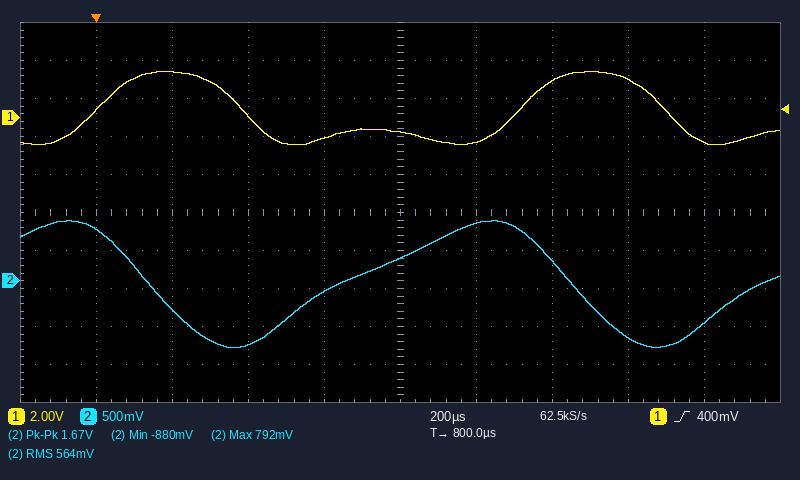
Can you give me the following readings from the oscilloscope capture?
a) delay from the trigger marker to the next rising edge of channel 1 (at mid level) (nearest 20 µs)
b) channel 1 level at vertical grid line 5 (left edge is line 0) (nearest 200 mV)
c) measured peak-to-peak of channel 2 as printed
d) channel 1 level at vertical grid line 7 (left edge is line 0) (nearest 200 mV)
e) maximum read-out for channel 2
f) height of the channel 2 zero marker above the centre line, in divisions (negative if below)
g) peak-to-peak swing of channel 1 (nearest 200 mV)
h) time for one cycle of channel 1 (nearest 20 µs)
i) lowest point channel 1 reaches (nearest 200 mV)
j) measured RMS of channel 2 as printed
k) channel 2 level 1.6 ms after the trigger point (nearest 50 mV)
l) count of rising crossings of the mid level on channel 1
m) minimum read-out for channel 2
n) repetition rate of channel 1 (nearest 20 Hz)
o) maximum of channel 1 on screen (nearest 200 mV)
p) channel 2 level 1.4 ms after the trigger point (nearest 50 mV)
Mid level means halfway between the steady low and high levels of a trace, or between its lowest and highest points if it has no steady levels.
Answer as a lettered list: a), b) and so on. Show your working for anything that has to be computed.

a) 1.12 ms
b) -800 mV
c) 1.67 V
d) 2.0 V
e) 792 mV
f) -1.8 div
g) 2.4 V − (-1.4 V) = 3.8 V
h) 1.12 ms
i) -1.4 V
j) 564 mV
k) -550 mV
l) 2
m) -880 mV
n) 1 / 1.12 ms ≈ 893 Hz, so 900 Hz to the nearest 20 Hz
o) 2.4 V
p) -750 mV
